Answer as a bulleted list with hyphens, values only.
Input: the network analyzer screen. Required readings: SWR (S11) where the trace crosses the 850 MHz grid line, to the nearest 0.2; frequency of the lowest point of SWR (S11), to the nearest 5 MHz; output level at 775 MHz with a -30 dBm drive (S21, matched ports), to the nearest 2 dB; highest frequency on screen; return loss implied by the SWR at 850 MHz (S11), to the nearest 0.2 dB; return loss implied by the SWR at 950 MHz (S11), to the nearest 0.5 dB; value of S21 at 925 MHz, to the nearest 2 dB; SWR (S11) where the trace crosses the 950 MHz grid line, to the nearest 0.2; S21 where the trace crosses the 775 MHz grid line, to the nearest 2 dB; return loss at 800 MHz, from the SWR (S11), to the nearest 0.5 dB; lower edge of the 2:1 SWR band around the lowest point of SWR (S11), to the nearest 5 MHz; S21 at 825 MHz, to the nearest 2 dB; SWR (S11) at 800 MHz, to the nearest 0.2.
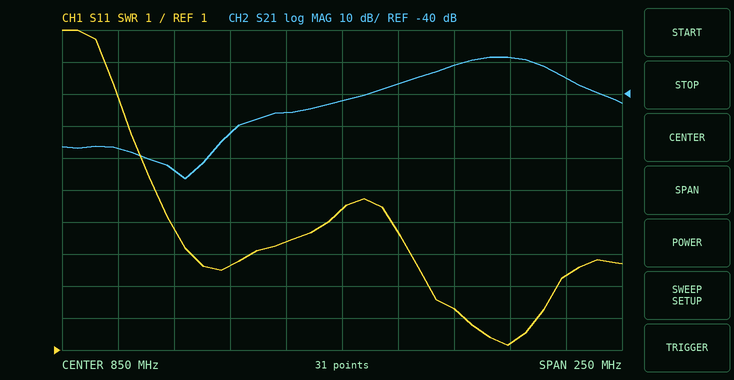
- 5.4
- 925 MHz
- -94 dBm
- 975 MHz
- 3.2 dB
- 5.5 dB
- -28 dB
- 3.4
- -64 dB
- 5.0 dB
- 905 MHz
- -46 dB
- 3.6
